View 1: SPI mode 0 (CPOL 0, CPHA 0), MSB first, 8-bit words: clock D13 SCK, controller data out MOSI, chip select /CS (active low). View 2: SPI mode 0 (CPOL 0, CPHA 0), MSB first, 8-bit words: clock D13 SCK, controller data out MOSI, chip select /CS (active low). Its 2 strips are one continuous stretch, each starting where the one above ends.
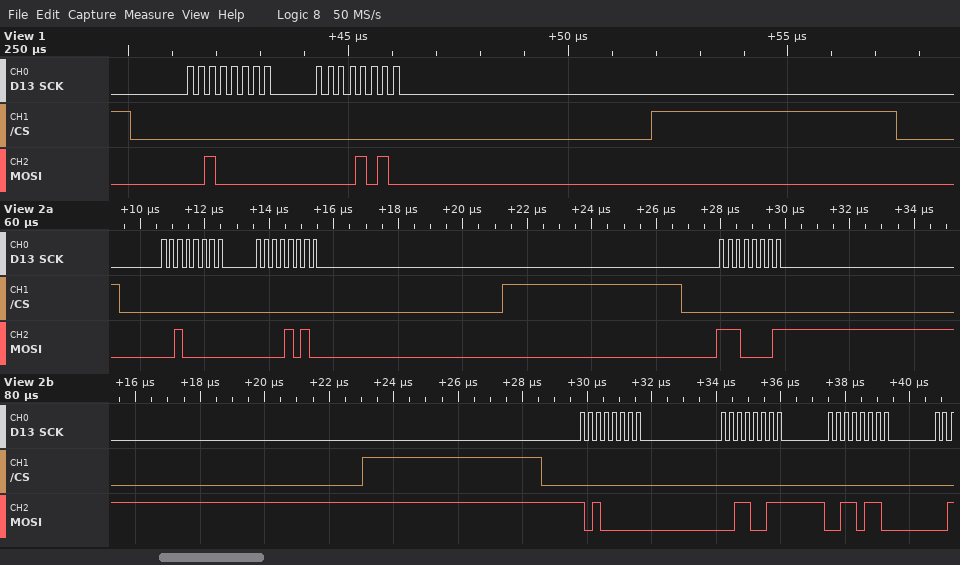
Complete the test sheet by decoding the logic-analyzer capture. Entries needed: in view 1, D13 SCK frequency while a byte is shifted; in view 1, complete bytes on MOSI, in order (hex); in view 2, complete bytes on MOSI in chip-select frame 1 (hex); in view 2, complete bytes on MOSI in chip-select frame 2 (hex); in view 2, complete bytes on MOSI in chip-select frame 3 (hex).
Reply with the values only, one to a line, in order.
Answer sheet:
4 MHz
20 0A
0x20 0x0A
0xE1
0xA0 0x33 0x36
